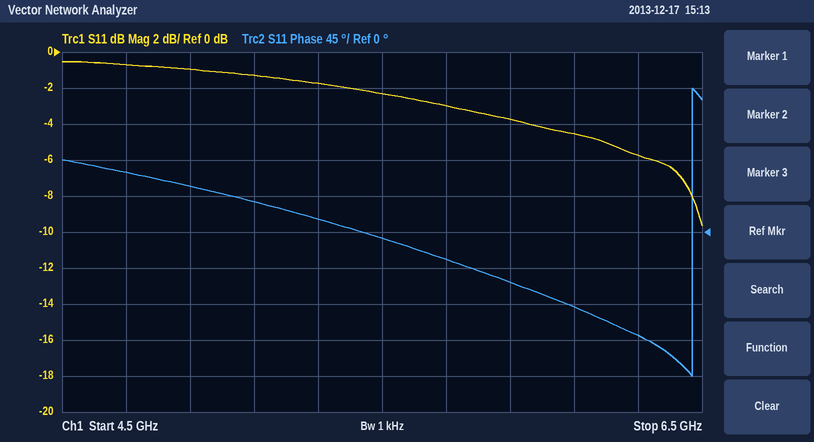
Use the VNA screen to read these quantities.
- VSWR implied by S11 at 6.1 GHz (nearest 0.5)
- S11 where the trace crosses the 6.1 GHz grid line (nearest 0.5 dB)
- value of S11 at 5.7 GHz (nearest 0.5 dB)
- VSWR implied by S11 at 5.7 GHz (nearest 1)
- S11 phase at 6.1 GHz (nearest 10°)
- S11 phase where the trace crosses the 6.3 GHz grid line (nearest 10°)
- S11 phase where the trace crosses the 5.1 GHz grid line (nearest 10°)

4.0
-4.5 dB
-3.0 dB
6
-90°
-130°
40°
